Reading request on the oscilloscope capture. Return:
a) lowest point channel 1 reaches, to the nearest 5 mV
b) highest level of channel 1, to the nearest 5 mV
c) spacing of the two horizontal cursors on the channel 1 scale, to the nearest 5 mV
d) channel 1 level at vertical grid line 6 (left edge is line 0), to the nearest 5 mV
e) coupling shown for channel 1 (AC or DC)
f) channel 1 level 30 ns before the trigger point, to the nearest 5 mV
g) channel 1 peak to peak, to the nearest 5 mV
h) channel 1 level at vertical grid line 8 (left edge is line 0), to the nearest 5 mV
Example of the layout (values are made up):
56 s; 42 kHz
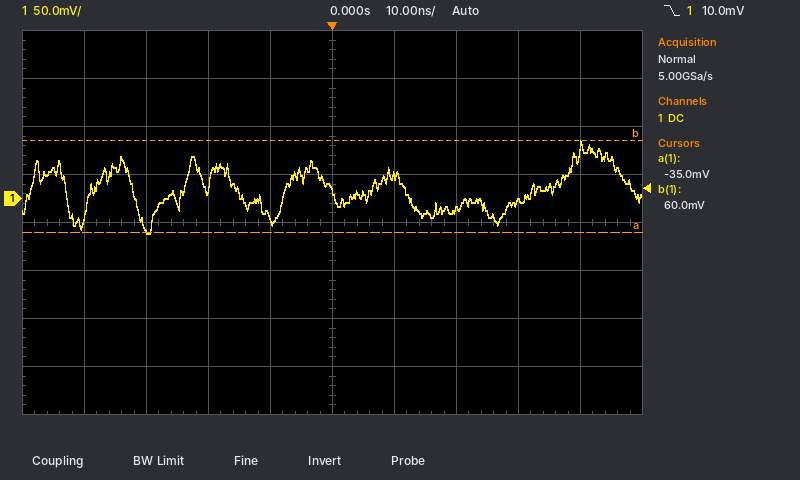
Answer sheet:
-35 mV; 60 mV; 95 mV; 25 mV; DC; -30 mV; 95 mV; -5 mV
